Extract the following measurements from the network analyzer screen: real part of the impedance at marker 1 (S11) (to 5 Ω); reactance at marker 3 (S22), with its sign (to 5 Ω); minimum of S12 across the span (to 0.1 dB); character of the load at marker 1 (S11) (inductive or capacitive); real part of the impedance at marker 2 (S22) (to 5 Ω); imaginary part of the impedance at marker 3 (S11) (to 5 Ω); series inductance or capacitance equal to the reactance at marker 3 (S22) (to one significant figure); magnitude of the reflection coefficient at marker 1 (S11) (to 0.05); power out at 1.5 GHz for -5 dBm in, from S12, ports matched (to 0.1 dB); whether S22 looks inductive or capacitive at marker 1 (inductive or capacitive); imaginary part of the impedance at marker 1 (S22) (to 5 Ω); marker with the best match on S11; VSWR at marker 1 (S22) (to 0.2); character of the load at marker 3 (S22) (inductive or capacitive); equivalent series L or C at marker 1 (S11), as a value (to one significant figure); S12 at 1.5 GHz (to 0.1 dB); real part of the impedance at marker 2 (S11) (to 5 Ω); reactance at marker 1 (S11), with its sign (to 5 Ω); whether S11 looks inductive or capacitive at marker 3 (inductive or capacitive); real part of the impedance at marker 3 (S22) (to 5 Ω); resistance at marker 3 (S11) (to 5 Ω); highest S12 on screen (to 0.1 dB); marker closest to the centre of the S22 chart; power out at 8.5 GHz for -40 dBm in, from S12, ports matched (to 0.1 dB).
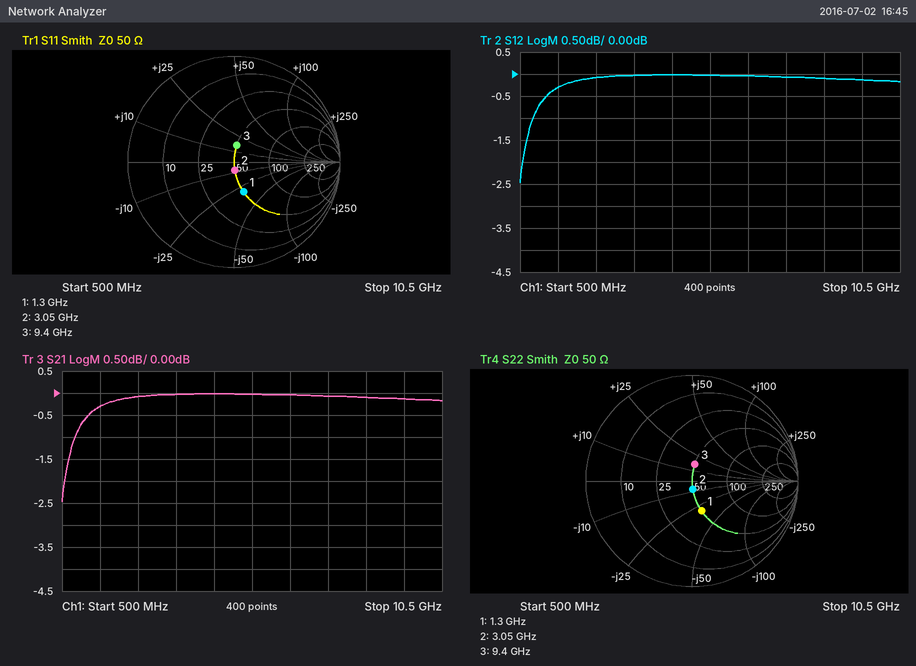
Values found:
50 Ω
+15 Ω
-2.5 dB
capacitive
50 Ω
+15 Ω
300 pH
0.30
-5.3 dBm
capacitive
-30 Ω
marker 2
1.8
inductive
4 pF
-0.3 dB
50 Ω
-30 Ω
inductive
50 Ω
50 Ω
0.0 dB
marker 2
-40.1 dBm
